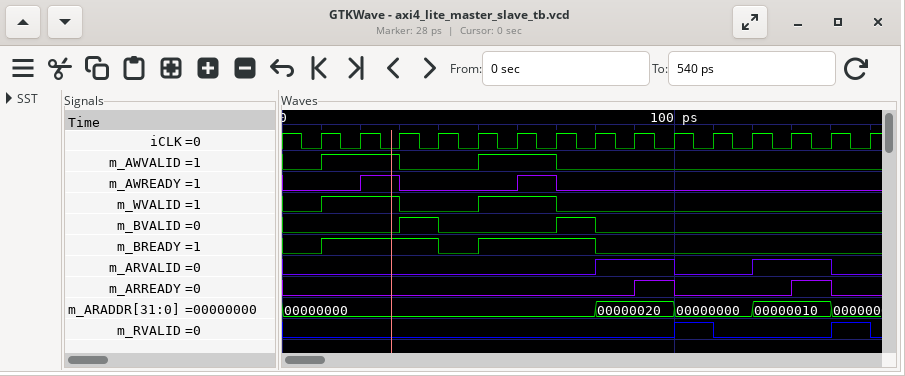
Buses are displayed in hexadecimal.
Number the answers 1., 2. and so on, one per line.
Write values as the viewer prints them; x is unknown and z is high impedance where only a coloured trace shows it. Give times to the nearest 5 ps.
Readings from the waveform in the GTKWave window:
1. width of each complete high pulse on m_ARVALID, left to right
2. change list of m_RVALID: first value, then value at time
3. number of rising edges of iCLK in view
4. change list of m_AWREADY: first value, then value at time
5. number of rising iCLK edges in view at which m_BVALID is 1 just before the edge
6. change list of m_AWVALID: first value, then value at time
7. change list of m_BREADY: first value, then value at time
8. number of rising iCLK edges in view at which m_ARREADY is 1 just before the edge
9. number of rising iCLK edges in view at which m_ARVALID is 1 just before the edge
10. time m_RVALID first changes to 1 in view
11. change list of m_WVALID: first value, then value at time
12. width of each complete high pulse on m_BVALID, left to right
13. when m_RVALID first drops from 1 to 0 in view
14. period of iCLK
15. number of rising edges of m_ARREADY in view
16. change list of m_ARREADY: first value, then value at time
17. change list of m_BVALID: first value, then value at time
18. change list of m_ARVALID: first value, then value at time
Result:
1. 20 ps, 20 ps
2. 0, 1 at 100 ps, 0 at 110 ps, 1 at 140 ps, 0 at 150 ps
3. 15
4. 0, 1 at 20 ps, 0 at 30 ps, 1 at 60 ps, 0 at 70 ps
5. 2
6. 0, 1 at 10 ps, 0 at 30 ps, 1 at 50 ps, 0 at 70 ps
7. 0, 1 at 10 ps, 0 at 40 ps, 1 at 50 ps, 0 at 80 ps
8. 2
9. 4
10. 100 ps
11. 0, 1 at 10 ps, 0 at 30 ps, 1 at 50 ps, 0 at 70 ps
12. 10 ps, 10 ps
13. 110 ps
14. 10 ps
15. 2
16. 0, 1 at 90 ps, 0 at 100 ps, 1 at 130 ps, 0 at 140 ps
17. 0, 1 at 30 ps, 0 at 40 ps, 1 at 70 ps, 0 at 80 ps
18. 0, 1 at 80 ps, 0 at 100 ps, 1 at 120 ps, 0 at 140 ps
